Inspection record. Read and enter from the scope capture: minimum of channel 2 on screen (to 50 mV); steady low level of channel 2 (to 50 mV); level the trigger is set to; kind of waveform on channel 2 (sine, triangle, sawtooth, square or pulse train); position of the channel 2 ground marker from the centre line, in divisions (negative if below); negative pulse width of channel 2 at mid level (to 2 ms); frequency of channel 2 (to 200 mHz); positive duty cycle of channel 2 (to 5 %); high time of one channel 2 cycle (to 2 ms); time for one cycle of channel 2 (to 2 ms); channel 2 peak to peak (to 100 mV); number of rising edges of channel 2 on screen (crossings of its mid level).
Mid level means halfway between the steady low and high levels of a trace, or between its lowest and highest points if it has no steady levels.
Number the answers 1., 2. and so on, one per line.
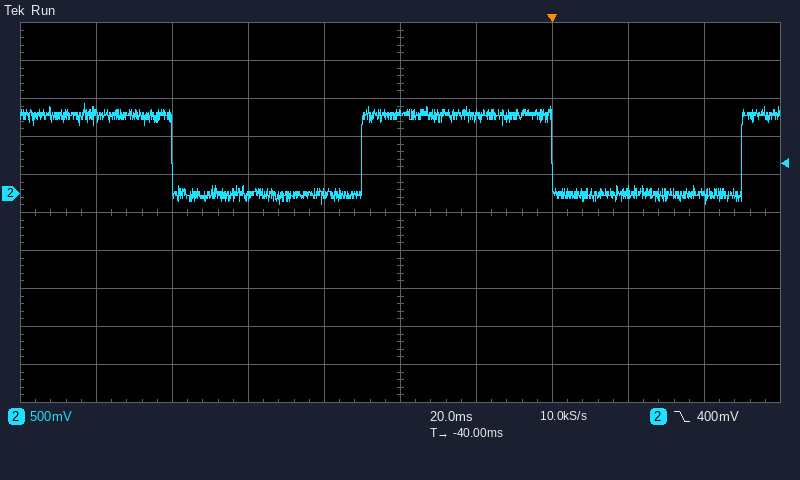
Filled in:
1. -150 mV
2. 0 mV
3. 400 mV
4. square
5. +0.5 div
6. 50 ms
7. 10.0 Hz
8. 50 %
9. 50 ms
10. 100 ms
11. 1.30 V
12. 2
